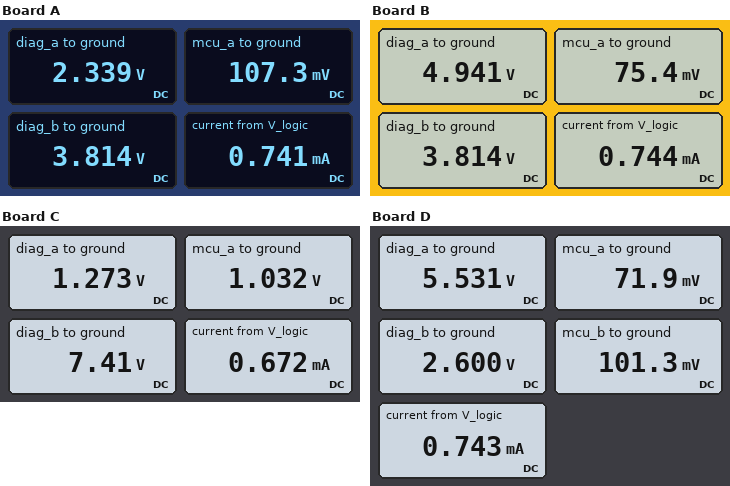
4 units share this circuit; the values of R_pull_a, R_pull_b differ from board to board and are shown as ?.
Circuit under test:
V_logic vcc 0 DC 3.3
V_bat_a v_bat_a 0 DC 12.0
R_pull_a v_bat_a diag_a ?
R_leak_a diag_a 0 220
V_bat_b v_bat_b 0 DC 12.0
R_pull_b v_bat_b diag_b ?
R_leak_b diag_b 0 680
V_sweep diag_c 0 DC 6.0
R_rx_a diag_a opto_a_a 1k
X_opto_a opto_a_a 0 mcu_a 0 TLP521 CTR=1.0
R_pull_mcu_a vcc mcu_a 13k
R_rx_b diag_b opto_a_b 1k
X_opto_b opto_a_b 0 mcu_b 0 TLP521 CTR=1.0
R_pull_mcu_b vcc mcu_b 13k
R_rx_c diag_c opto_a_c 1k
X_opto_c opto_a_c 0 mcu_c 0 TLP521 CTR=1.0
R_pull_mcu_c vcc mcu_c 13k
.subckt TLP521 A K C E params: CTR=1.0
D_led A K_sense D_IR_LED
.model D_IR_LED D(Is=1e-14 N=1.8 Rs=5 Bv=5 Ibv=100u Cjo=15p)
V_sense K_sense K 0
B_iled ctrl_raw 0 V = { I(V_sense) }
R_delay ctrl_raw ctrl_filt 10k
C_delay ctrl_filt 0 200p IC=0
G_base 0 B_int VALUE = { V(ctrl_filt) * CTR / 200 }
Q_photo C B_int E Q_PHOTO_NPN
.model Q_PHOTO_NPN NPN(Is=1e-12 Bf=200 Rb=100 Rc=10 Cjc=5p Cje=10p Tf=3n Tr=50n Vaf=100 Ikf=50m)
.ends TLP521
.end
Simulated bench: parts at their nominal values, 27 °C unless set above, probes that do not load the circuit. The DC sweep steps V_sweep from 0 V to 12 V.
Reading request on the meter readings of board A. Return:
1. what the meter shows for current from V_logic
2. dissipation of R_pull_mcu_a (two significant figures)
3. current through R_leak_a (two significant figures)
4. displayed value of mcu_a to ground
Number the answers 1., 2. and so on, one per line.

1. 0.741 mA
2. 780 µW
3. 11 mA
4. 107.3 mV
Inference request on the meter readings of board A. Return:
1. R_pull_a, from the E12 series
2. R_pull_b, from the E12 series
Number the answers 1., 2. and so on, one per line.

1. 820 Ω
2. 1 kΩ
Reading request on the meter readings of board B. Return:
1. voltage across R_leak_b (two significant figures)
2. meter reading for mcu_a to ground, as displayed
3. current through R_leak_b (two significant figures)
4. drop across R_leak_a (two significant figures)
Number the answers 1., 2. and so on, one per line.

1. 3.8 V
2. 75.4 mV
3. 5.6 mA
4. 4.9 V
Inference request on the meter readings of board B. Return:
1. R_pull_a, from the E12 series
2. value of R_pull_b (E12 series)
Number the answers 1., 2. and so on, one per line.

1. 270 Ω
2. 1 kΩ
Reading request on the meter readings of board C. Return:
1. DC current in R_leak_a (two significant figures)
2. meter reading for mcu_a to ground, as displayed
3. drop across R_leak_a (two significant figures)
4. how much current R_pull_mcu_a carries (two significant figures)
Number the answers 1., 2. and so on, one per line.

1. 5.8 mA
2. 1.032 V
3. 1.3 V
4. 170 µA
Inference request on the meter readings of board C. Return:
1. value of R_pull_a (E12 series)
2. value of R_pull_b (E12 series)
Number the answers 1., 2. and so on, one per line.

1. 1.8 kΩ
2. 270 Ω
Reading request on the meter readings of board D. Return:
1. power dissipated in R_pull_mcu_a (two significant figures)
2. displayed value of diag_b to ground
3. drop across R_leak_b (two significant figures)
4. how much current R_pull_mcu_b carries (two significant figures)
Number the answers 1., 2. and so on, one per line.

1. 800 µW
2. 2.600 V
3. 2.6 V
4. 250 µA
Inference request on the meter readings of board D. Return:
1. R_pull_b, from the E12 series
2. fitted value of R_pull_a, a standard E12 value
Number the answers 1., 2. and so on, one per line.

1. 1.8 kΩ
2. 220 Ω
